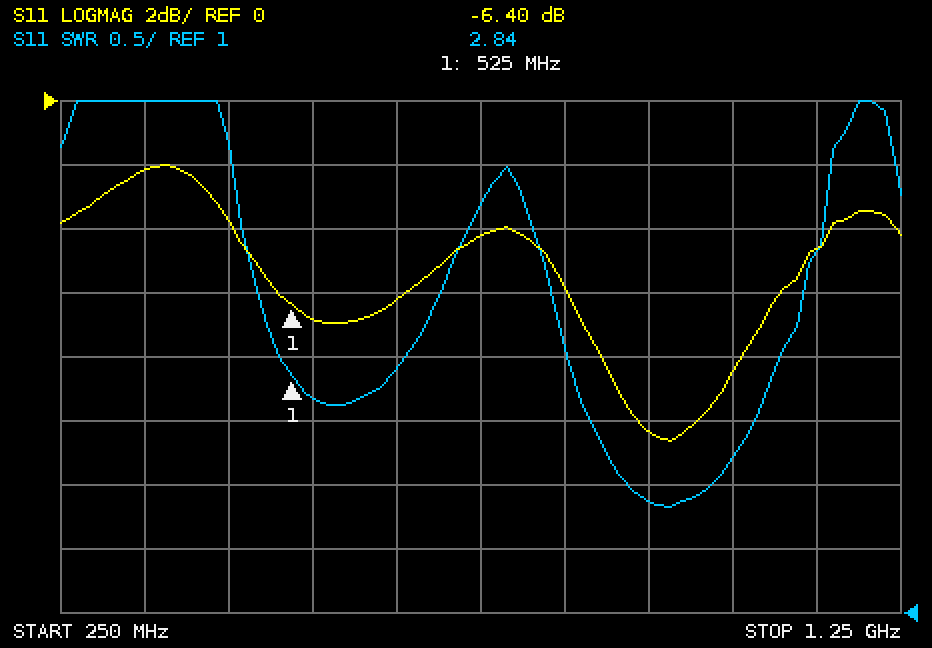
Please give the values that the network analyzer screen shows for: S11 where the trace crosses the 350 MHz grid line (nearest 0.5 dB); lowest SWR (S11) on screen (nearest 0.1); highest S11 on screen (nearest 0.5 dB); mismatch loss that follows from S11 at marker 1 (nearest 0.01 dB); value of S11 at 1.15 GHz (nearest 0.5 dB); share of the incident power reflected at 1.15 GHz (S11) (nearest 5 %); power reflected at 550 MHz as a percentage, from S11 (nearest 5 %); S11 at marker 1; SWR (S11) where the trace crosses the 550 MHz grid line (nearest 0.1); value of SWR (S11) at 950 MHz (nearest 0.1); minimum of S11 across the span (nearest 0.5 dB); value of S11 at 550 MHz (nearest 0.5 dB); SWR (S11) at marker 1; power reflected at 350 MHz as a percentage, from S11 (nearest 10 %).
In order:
-2.0 dB
1.8
-2.0 dB
1.13 dB
-4.5 dB
35 %
20 %
-6.40 dB
2.7
1.9
-10.5 dB
-7.0 dB
2.84
60 %
